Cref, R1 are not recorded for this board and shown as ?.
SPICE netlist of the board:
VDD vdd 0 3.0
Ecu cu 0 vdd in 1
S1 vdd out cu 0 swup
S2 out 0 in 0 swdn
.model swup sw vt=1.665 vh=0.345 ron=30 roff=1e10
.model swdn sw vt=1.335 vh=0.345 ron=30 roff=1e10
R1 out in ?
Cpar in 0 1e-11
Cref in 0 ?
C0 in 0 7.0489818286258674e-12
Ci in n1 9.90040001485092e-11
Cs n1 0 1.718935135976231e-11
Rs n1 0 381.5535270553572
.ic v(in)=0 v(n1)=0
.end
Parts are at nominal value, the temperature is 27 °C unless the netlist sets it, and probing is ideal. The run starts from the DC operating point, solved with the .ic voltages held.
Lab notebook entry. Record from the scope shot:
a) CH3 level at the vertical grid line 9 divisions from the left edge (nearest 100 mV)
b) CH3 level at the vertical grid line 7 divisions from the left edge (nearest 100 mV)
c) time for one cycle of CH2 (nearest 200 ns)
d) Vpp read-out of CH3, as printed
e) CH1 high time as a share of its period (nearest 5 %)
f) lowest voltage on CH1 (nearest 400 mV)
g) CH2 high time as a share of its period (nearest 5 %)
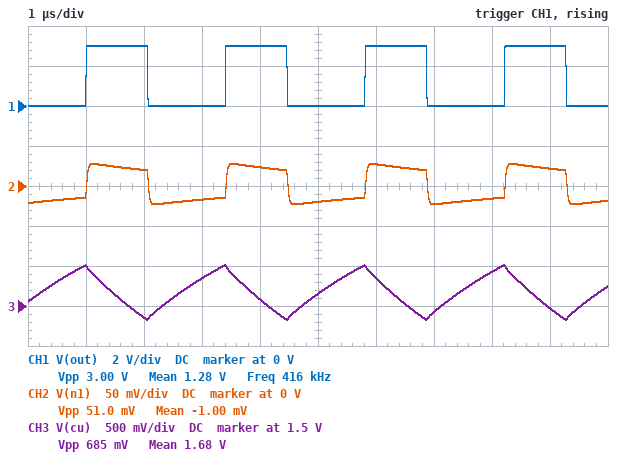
1.5 V
1.4 V
2.4 µs
685 mV
45 %
0 V
45 %
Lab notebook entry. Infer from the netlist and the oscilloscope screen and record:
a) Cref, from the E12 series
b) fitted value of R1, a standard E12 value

56 pF
15 kΩ
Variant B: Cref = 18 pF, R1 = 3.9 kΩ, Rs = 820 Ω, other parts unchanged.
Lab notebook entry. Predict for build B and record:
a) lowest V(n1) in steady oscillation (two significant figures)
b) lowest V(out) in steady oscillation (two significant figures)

-170 mV
7.6 mV
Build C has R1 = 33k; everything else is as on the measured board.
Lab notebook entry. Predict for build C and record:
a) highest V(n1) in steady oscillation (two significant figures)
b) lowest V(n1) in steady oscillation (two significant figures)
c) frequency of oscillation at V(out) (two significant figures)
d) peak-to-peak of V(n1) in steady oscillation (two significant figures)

13 mV
-11 mV
190 kHz
24 mV
